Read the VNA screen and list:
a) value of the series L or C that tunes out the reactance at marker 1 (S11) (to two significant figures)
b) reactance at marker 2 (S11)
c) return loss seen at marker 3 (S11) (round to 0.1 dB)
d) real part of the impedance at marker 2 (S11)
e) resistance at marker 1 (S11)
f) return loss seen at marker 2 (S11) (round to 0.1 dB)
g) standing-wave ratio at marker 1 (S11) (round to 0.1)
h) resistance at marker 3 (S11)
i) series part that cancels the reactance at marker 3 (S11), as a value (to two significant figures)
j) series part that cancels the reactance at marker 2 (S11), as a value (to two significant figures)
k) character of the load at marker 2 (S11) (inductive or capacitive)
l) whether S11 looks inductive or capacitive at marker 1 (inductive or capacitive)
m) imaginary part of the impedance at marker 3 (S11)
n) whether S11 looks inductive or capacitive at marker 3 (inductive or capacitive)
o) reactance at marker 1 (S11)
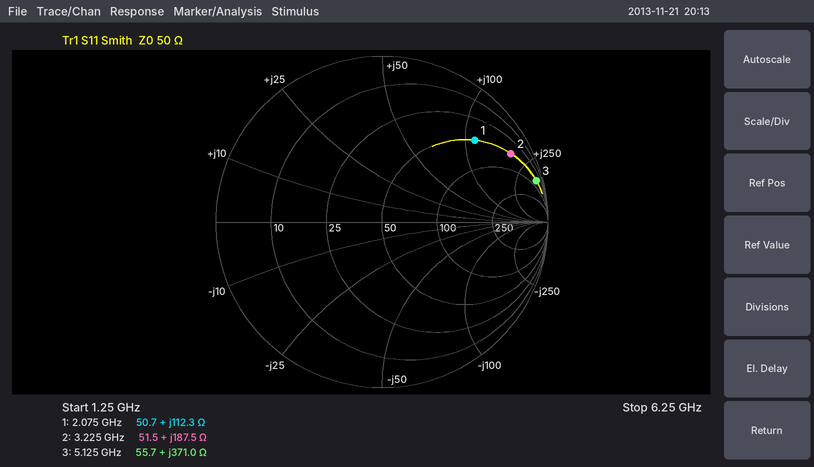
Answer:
680 fF
+187.5 Ω
0.3 dB
51.5 Ω
50.7 Ω
1.1 dB
6.8
55.7 Ω
84 fF
260 fF
inductive
inductive
+371.0 Ω
inductive
+112.3 Ω
